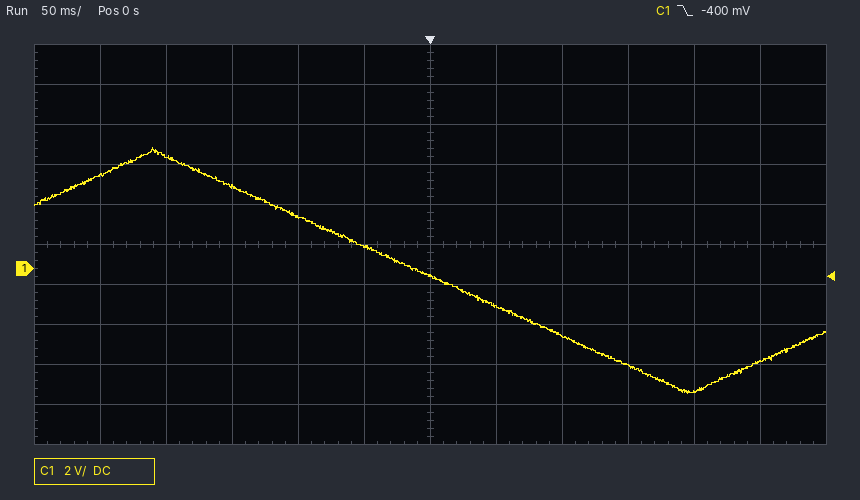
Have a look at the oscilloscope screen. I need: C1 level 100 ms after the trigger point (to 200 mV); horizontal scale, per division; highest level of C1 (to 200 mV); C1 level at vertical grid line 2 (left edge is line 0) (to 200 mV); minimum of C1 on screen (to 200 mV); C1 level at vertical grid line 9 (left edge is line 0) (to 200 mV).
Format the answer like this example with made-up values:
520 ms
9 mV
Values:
-3.4 V
50 ms
6.0 V
5.6 V
-6.2 V
-4.8 V
